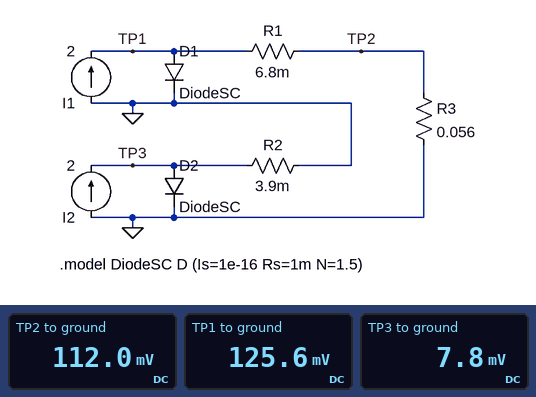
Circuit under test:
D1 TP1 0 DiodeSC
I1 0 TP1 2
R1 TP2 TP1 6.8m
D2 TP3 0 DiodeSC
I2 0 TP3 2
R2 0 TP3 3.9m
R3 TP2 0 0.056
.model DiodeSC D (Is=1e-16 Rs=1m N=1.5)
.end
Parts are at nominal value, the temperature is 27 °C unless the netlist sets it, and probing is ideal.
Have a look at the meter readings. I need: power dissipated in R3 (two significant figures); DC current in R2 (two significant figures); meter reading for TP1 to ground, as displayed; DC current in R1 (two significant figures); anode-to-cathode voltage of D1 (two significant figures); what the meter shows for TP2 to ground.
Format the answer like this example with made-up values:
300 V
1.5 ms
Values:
220 mW
2.0 A
125.6 mV
2.0 A
130 mV
112.0 mV
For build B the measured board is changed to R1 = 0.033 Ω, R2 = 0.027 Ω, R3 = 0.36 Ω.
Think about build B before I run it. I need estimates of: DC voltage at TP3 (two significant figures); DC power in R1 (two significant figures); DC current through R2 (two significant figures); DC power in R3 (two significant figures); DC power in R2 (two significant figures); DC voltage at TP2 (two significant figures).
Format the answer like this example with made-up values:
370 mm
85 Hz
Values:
54 mV
130 mW
2.0 A
1.4 W
110 mW
720 mV
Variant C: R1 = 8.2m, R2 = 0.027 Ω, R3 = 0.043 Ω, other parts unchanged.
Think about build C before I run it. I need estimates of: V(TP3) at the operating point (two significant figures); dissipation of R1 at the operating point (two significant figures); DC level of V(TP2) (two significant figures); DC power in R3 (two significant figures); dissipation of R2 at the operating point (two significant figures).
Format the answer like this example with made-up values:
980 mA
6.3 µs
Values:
54 mV
33 mW
86 mV
170 mW
110 mW
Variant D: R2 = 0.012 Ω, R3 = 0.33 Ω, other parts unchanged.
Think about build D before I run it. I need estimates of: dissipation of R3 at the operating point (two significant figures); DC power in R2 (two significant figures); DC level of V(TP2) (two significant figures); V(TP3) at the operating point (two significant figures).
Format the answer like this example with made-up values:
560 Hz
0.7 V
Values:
1.3 W
48 mW
660 mV
24 mV
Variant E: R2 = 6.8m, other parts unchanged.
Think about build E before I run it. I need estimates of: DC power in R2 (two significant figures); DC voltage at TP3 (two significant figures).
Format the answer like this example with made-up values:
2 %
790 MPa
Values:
27 mW
14 mV
